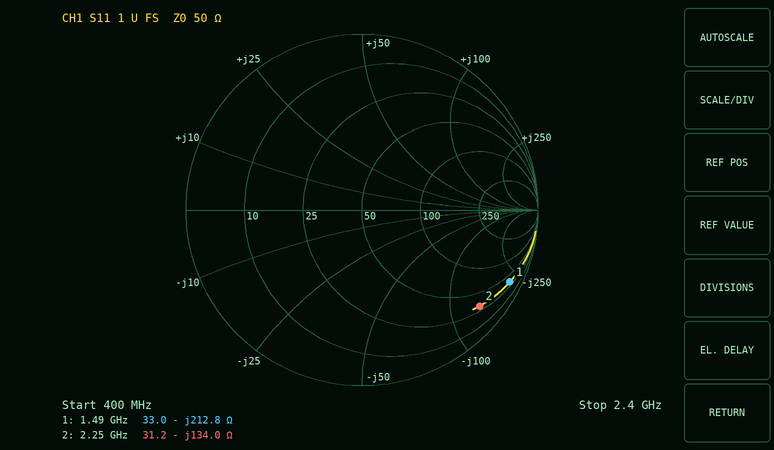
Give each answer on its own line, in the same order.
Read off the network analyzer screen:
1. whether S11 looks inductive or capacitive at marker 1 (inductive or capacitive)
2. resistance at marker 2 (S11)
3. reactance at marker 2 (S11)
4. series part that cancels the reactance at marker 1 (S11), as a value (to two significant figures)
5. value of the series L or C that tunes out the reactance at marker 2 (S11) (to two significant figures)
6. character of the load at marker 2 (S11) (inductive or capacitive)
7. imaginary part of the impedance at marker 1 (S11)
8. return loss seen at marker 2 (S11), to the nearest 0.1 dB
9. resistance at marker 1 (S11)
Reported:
capacitive
31.2 Ω
-134.0 Ω
23 nH
9.5 nH
capacitive
-212.8 Ω
1.3 dB
33.0 Ω
